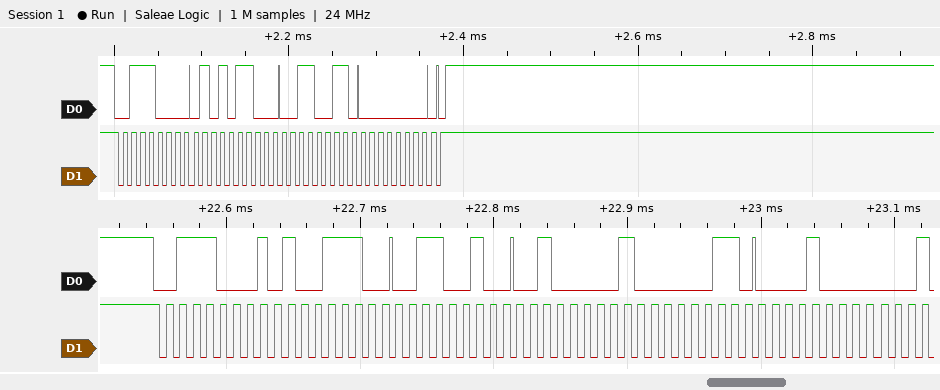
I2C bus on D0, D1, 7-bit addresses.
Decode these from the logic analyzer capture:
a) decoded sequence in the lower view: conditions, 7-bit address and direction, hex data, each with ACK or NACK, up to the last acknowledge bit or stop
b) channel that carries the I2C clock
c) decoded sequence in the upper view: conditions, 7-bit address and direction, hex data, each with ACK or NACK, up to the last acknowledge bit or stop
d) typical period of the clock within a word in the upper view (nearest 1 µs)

start, address 38 read ACK, 9C ACK, 64 ACK, 41 ACK, 06 ACK, 10 ACK
D1
start, address 38 write ACK, AC ACK, 33 ACK, 00 ACK, stop
10 µs
